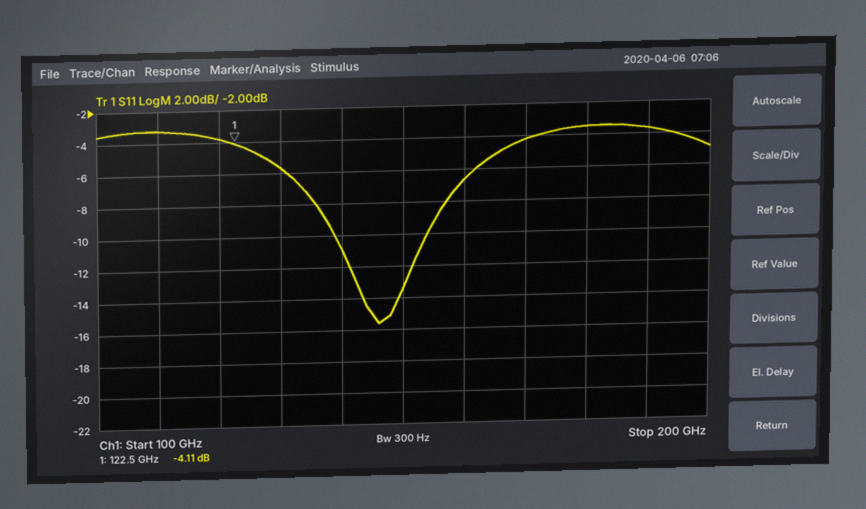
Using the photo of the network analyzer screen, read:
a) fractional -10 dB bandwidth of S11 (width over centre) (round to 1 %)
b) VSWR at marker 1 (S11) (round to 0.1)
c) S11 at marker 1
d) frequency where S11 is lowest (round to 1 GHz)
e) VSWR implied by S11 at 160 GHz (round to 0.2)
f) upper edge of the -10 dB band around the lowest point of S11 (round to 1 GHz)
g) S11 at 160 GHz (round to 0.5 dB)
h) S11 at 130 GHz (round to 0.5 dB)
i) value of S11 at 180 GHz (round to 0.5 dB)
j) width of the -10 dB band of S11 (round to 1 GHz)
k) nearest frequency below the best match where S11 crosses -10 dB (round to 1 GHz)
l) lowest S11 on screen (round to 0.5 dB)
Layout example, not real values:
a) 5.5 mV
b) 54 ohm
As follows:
a) 10 %
b) 4.3
c) -4.11 dB
d) 146 GHz
e) 2.8
f) 154 GHz
g) -6.5 dB
h) -5.5 dB
i) -3.5 dB
j) 15 GHz
k) 139 GHz
l) -15.5 dB
